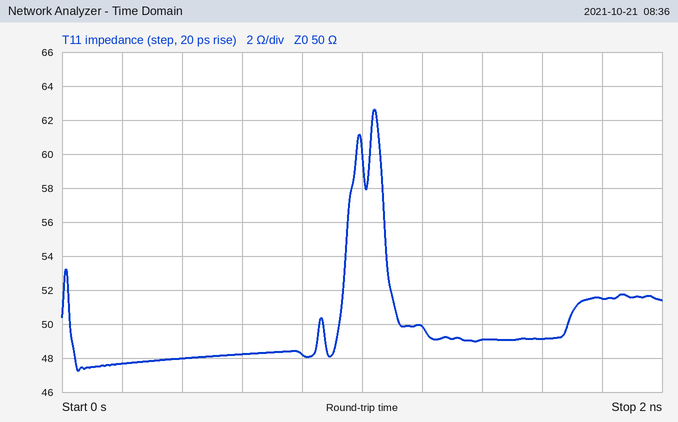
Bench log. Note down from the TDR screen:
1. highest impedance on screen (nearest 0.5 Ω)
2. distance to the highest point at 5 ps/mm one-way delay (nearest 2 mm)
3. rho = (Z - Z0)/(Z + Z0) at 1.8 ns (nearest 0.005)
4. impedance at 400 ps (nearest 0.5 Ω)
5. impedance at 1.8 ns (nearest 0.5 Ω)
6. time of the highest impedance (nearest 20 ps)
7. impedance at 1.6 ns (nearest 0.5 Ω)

62.5 Ω
104 mm
+0.015
48.0 Ω
51.5 Ω
1.04 ns
49.0 Ω
